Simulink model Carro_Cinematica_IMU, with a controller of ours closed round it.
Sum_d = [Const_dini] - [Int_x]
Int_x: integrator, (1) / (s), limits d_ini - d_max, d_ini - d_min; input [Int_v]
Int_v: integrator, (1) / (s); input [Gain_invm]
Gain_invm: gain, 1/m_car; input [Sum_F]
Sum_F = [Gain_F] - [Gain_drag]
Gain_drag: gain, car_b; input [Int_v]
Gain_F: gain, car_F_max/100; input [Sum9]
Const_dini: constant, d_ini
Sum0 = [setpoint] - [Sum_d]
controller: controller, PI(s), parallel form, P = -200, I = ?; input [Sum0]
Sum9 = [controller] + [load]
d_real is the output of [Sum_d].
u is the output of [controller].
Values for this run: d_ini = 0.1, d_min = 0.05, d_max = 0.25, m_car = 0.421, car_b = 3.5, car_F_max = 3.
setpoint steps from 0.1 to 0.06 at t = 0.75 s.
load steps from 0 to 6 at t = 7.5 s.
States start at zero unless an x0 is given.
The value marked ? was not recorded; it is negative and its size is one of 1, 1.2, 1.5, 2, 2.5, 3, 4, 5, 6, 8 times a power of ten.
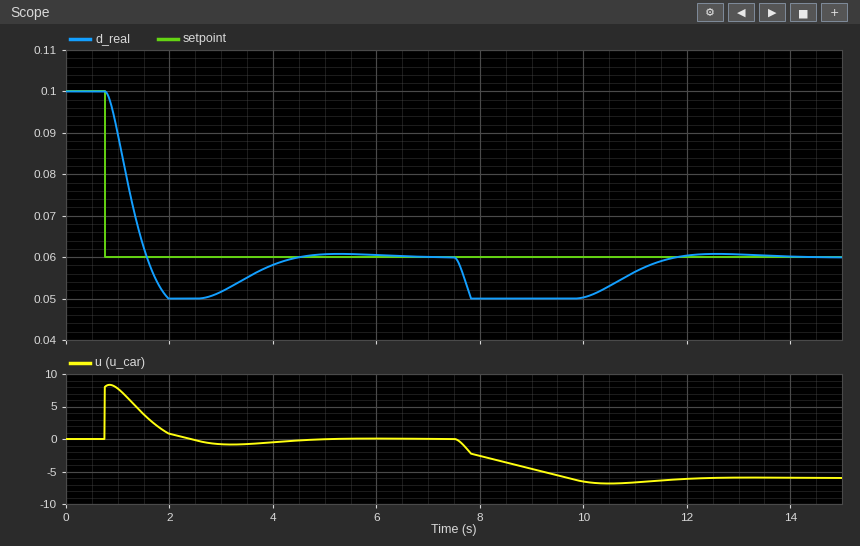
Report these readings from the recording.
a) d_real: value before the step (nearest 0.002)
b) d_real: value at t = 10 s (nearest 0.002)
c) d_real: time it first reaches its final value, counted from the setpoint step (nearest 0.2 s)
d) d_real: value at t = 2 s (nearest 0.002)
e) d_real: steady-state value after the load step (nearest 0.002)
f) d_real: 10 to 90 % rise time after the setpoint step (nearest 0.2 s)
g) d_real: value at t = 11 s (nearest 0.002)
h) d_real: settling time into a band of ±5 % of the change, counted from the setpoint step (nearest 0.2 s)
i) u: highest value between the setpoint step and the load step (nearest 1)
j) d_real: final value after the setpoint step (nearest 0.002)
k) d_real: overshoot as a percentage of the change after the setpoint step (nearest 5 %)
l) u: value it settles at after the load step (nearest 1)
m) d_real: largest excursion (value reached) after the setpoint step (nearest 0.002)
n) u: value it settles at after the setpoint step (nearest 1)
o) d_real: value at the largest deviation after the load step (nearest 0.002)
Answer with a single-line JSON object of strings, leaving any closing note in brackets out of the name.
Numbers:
{"d_real: value before the step": "0.100", "d_real: value at t = 10 s": "0.050", "d_real: time it first reaches its final value, counted from the setpoint step": "0.8 s", "d_real: value at t = 2 s": "0.050", "d_real: steady-state value after the load step": "0.060", "d_real: 10 to 90 % rise time after the setpoint step": "0.6 s", "d_real: value at t = 11 s": "0.056", "d_real: settling time into a band of ±5 % of the change, counted from the setpoint step": "3.2 s", "u: highest value between the setpoint step and the load step": "8", "d_real: final value after the setpoint step": "0.060", "d_real: overshoot as a percentage of the change after the setpoint step": "25 %", "u: value it settles at after the load step": "-6", "d_real: largest excursion (value reached) after the setpoint step": "0.050", "u: value it settles at after the setpoint step": "0", "d_real: value at the largest deviation after the load step": "0.050"}
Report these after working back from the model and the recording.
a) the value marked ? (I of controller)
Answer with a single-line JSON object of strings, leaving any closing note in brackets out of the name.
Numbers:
{"the value marked ?": "-200"}
